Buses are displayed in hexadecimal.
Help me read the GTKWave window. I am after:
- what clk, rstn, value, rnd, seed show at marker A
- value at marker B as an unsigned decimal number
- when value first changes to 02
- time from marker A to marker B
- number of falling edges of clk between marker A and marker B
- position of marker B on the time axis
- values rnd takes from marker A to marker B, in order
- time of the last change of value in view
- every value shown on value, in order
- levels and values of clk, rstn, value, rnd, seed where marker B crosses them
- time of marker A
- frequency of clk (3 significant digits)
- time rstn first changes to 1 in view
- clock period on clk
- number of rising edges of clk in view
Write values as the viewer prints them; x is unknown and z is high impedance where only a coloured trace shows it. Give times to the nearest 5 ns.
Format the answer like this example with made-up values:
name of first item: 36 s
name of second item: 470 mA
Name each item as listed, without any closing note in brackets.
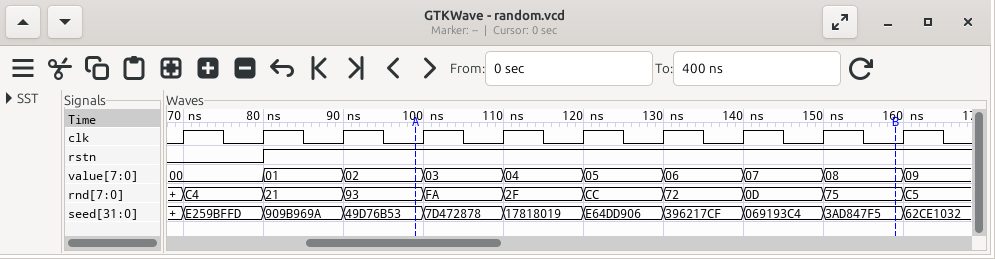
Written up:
what clk, rstn, value, rnd, seed show at marker A: clk=0, rstn=1, value=02, rnd=93, seed=49D76B53
value at marker B as an unsigned decimal number: 8
when value first changes to 02: 90 ns
time from marker A to marker B: 60 ns
number of falling edges of clk between marker A and marker B: 6
position of marker B on the time axis: 160 ns
values rnd takes from marker A to marker B, in order: 93, FA, 2F, CC, 72, 0D, 75
time of the last change of value in view: 160 ns
every value shown on value, in order: 00, 01, 02, 03, 04, 05, 06, 07, 08, 09
levels and values of clk, rstn, value, rnd, seed where marker B crosses them: clk=0, rstn=1, value=08, rnd=75, seed=3AD847F5
time of marker A: 100 ns
frequency of clk: 100 MHz
time rstn first changes to 1 in view: 80 ns
clock period on clk: 10 ns
number of rising edges of clk in view: 10
